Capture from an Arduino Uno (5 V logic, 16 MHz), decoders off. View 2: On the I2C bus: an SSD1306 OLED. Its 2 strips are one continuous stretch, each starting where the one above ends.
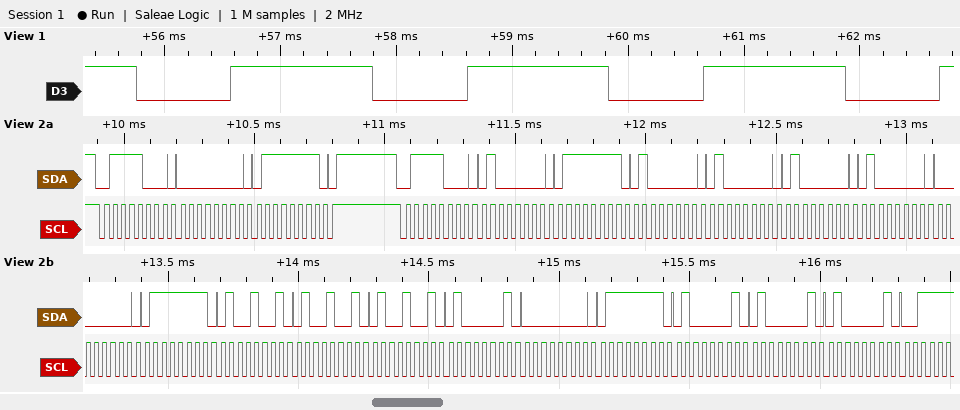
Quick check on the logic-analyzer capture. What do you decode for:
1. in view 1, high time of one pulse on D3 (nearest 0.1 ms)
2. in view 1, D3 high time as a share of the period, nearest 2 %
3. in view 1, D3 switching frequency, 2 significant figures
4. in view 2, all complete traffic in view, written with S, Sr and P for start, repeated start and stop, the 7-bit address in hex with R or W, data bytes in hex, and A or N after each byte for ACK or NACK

1.2 ms
60 %
490 Hz
S 3CW A 00 A 7F A P S 3CW A 40 A 7F A 40 A 40 A 40 A 40 A 00 A 7F A 49 A 49 A 49 A 41 A 00 A 7F A 41 A 41 A 41 A
